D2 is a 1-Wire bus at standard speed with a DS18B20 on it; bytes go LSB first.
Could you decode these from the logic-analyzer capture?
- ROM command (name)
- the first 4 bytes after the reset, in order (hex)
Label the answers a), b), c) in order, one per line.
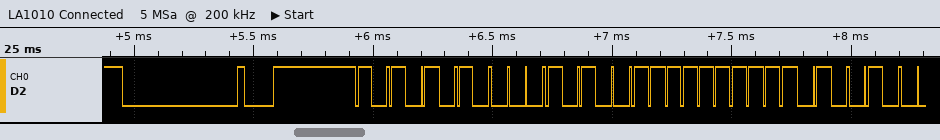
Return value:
a) Match ROM
b) 55 28 FF 4B
